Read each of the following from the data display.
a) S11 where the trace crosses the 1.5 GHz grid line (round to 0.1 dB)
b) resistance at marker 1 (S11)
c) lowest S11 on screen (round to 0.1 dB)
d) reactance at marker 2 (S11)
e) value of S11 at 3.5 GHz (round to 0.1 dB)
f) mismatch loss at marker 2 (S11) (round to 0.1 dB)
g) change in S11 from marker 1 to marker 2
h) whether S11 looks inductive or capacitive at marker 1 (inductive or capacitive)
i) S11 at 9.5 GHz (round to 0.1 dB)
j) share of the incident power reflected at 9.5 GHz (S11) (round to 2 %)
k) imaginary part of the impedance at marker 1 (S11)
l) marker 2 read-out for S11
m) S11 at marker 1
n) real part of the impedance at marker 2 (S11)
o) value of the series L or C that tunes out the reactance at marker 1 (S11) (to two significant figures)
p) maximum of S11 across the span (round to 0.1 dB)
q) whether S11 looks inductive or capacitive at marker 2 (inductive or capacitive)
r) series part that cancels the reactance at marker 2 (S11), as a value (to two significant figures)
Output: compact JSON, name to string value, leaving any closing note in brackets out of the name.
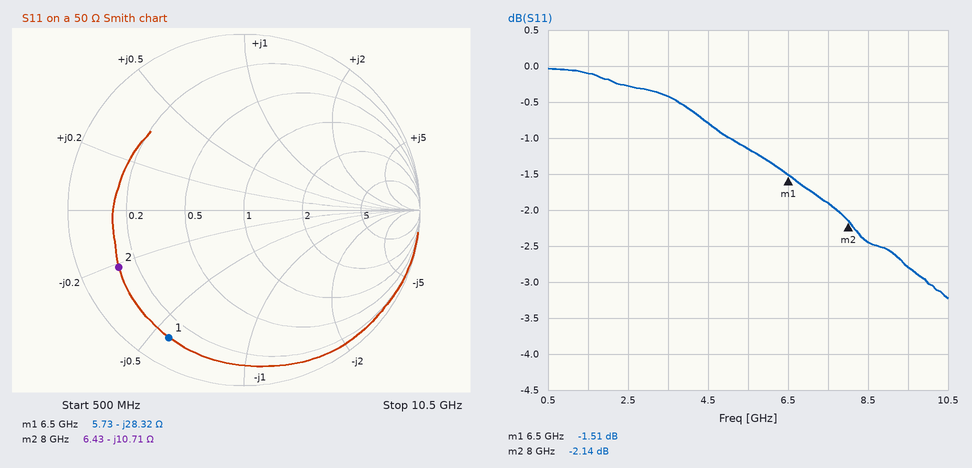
{"S11 where the trace crosses the 1.5 GHz grid line": "-0.1 dB", "resistance at marker 1": "5.73 Ω", "lowest S11 on screen": "-3.2 dB", "reactance at marker 2": "-10.71 Ω", "value of S11 at 3.5 GHz": "-0.4 dB", "mismatch loss at marker 2 (S11)": "4.1 dB", "change in S11 from marker 1 to marker 2": "-0.63 dB", "whether S11 looks inductive or capacitive at marker 1": "capacitive", "S11 at 9.5 GHz": "-2.8 dB", "share of the incident power reflected at 9.5 GHz (S11)": "52 %", "imaginary part of the impedance at marker 1": "-28.32 Ω", "marker 2 read-out for S11": "-2.14 dB", "S11 at marker 1": "-1.51 dB", "real part of the impedance at marker 2": "6.43 Ω", "value of the series L or C that tunes out the reactance at marker 1 (S11)": "690 pH", "maximum of S11 across the span": "0.0 dB", "whether S11 looks inductive or capacitive at marker 2": "capacitive", "series part that cancels the reactance at marker 2 (S11), as a value": "210 pH"}
